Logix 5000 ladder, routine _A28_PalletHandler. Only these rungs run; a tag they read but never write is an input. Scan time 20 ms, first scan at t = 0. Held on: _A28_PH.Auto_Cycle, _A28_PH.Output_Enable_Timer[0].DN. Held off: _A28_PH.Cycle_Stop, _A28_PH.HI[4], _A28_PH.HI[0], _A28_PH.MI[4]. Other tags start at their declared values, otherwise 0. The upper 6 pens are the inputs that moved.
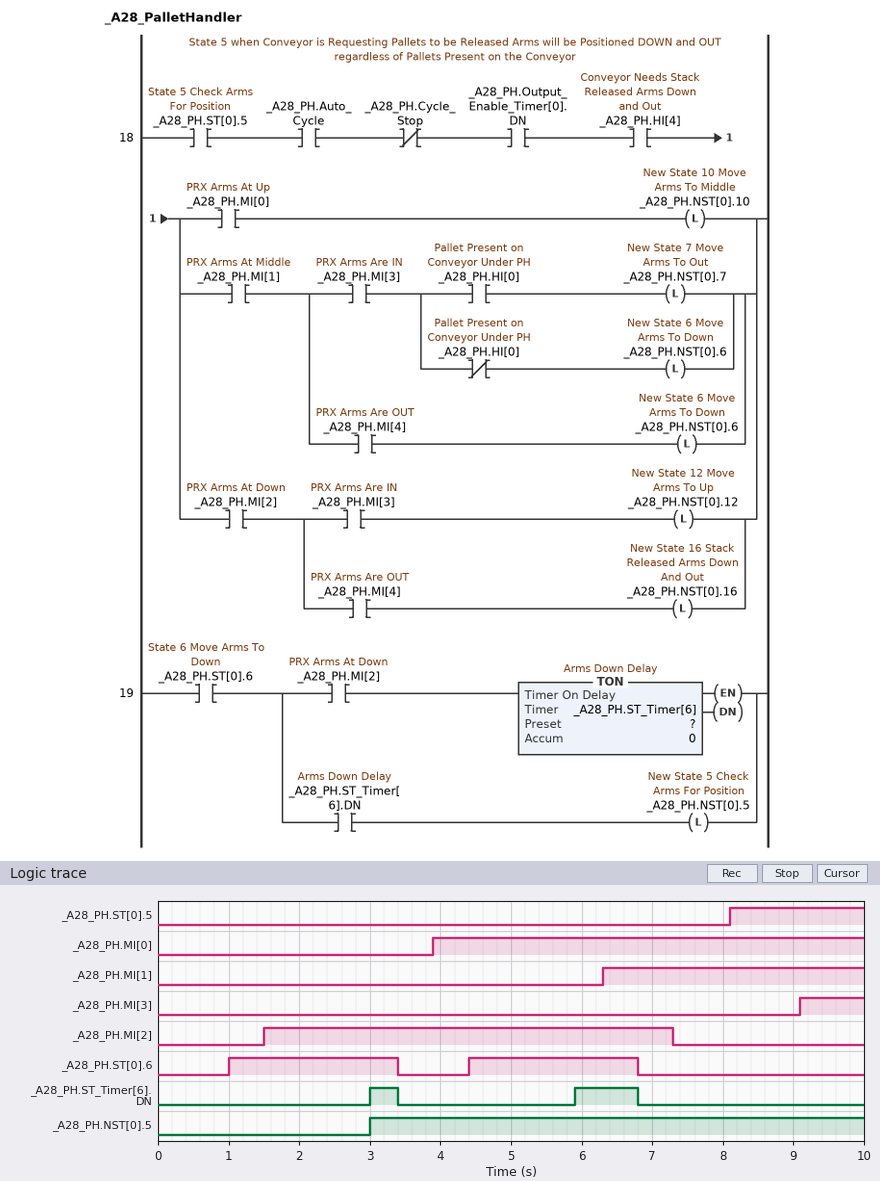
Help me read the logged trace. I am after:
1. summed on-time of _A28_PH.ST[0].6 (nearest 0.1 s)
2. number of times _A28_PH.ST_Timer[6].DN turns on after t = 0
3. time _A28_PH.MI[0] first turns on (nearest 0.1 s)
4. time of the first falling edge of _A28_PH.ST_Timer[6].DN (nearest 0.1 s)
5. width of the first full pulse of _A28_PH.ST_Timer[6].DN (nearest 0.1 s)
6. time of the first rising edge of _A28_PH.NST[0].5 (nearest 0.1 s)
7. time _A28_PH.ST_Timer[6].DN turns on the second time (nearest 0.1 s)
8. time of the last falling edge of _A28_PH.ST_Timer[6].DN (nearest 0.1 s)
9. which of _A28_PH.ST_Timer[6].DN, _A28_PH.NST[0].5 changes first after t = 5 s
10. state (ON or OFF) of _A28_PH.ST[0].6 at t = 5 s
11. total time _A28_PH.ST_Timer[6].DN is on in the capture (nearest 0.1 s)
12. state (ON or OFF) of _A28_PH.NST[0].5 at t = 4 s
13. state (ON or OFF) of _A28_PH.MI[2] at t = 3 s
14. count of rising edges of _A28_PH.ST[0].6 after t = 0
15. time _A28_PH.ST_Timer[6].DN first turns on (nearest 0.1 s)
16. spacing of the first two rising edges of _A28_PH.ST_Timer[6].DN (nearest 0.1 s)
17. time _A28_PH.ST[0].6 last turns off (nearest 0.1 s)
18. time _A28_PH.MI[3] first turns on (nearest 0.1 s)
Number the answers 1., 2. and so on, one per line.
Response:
1. 4.8 s
2. 2
3. 3.9 s
4. 3.4 s
5. 0.4 s
6. 3.0 s
7. 5.9 s
8. 6.8 s
9. _A28_PH.ST_Timer[6].DN
10. ON
11. 1.3 s
12. ON
13. ON
14. 2
15. 3.0 s
16. 2.9 s
17. 6.8 s
18. 9.1 s
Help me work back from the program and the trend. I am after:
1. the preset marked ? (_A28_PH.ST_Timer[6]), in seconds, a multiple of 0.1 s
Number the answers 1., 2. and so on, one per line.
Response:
1. 1.5 s
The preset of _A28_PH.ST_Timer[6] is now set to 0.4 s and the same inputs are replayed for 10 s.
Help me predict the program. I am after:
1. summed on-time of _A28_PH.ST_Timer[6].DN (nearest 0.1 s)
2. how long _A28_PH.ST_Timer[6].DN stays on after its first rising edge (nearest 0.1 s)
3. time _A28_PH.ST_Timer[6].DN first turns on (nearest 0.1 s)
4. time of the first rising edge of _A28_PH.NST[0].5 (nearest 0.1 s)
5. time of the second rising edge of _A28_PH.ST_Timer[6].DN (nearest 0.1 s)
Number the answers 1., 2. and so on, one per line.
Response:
1. 3.5 s
2. 1.5 s
3. 1.9 s
4. 1.9 s
5. 4.8 s
